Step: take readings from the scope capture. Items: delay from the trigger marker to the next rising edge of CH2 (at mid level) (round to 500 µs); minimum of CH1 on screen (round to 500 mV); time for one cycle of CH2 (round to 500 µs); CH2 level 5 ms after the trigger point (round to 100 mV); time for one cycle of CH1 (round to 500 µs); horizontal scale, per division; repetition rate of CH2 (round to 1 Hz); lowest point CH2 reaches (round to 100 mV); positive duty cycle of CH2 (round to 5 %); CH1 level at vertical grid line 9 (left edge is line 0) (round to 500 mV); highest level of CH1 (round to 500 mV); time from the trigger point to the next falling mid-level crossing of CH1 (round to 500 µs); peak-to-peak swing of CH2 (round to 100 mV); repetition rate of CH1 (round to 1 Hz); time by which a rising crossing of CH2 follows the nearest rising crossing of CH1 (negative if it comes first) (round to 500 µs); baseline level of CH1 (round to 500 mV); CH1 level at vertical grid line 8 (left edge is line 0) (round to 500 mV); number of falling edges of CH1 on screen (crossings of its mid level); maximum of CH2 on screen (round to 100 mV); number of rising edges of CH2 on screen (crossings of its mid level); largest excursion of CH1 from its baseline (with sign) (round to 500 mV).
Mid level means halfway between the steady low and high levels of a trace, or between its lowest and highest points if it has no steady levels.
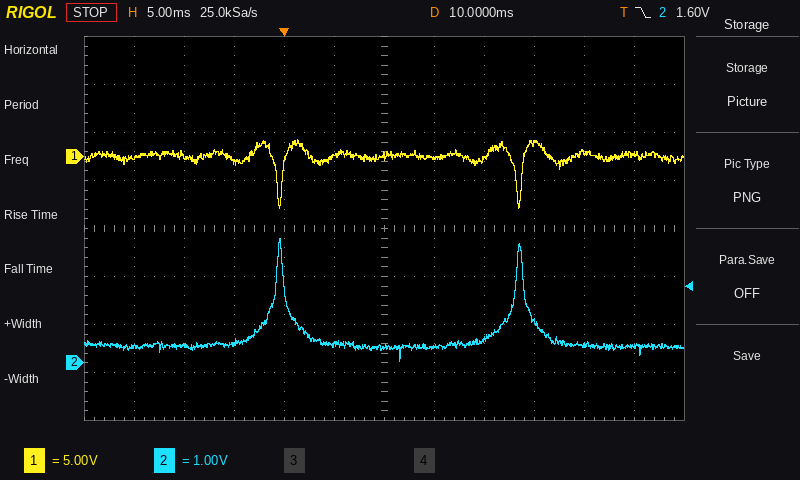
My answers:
23.0 ms
-5.5 V
24.0 ms
400 mV
24.0 ms
5 ms
42 Hz
0.0 V
5 %
1.5 V
2.0 V
23.0 ms
2.6 V
42 Hz
-1.0 ms
0.0 V
-500 mV
2
2.6 V
2
-5.5 V
